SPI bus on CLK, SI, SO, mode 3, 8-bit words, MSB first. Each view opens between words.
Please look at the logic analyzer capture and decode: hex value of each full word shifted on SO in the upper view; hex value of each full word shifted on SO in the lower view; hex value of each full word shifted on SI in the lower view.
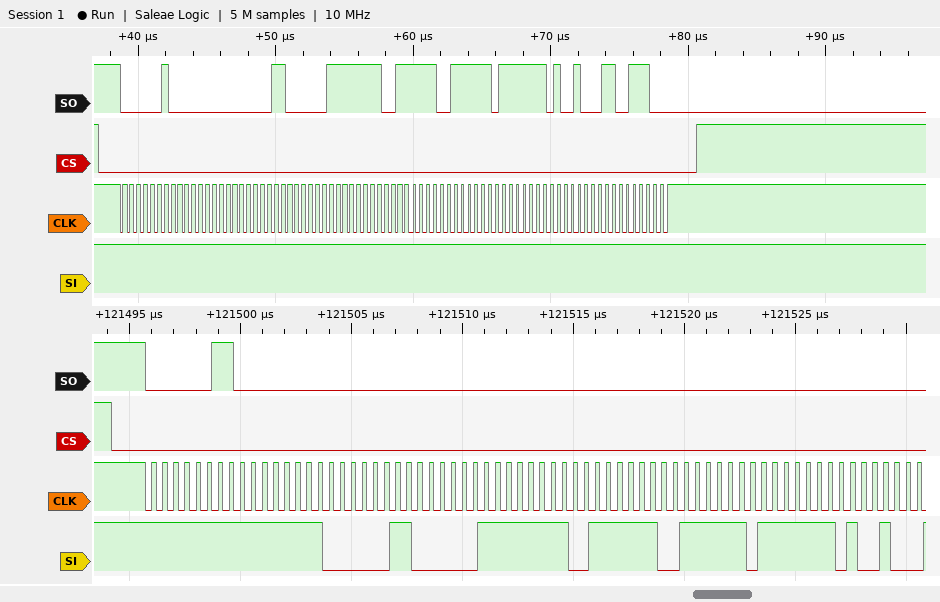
02, 00, 03, 03, FC, FC, FD, FD, 23, 38
03, 00, 00, 00, 00, 00, 00, 00
FF, FF, 03, 03, FC, FC, FD, FD
